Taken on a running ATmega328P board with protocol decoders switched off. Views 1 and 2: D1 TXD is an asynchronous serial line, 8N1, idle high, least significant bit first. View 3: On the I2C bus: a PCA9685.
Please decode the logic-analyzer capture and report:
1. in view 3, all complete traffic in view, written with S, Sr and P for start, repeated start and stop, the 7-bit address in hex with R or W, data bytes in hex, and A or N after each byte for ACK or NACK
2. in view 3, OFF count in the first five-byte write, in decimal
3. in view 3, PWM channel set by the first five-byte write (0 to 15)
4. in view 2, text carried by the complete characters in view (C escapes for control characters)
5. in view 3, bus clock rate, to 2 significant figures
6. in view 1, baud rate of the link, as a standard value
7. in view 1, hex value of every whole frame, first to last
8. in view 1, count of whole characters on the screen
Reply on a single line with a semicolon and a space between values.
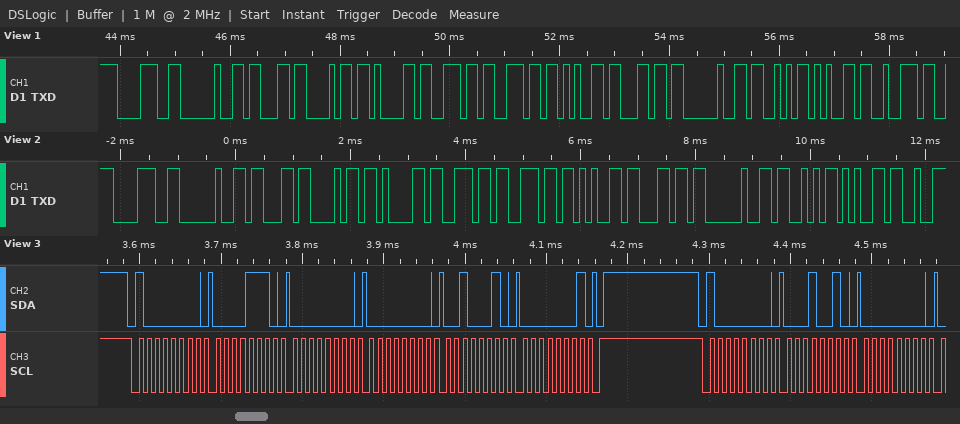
S 40W A 0E A 00 A 00 A 22 A 01 A P S 40W A 12 A 00 A; 290; 2; "8 channel Se"; 100 kHz; 9600 baud; 38 20 63 68 61 6E 6E 65 6C 20 53 65 72; 13
